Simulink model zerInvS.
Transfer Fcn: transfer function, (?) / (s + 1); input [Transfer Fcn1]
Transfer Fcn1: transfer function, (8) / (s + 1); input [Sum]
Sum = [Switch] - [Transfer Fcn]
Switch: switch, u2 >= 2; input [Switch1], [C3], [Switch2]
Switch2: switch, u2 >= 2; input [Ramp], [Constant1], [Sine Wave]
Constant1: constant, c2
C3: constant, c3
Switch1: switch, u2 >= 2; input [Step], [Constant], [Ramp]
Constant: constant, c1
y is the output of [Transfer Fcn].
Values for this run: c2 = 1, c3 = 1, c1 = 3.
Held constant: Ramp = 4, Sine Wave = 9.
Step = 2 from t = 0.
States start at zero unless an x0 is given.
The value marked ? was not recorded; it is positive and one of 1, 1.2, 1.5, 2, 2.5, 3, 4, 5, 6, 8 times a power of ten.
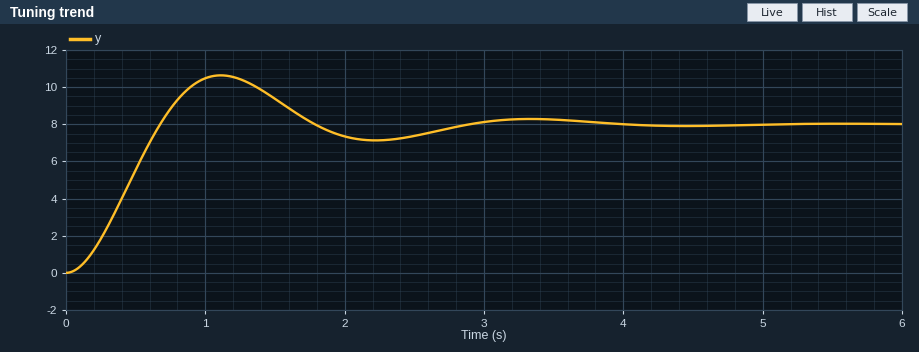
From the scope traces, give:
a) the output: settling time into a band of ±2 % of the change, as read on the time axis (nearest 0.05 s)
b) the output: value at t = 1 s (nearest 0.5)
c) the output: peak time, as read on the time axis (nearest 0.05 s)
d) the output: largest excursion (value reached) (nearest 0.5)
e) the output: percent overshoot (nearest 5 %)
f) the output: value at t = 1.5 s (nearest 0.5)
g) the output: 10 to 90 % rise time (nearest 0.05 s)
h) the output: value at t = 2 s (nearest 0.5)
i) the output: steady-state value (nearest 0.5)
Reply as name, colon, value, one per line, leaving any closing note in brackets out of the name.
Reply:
the output: settling time into a band of ±2 % of the change, as read on the time axis: 3.70 s
the output: value at t = 1 s: 10.5
the output: peak time, as read on the time axis: 1.10 s
the output: largest excursion (value reached): 10.5
the output: percent overshoot: 35 %
the output: value at t = 1.5 s: 9.5
the output: 10 to 90 % rise time: 0.45 s
the output: value at t = 2 s: 7.5
the output: steady-state value: 8.0
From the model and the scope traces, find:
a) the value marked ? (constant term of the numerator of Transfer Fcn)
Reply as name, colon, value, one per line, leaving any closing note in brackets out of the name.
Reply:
the value marked ?: 1
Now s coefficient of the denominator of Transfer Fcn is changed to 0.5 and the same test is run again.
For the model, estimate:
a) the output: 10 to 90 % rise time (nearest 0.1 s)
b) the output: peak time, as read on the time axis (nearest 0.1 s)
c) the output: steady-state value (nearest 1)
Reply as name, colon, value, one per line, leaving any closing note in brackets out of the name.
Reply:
the output: 10 to 90 % rise time: 0.3 s
the output: peak time, as read on the time axis: 0.8 s
the output: steady-state value: 8
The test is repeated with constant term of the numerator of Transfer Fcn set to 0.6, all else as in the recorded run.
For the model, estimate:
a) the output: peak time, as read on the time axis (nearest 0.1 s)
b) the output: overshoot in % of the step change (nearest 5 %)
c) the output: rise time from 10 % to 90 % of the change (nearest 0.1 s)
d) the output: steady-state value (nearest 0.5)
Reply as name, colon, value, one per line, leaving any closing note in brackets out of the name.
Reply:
the output: peak time, as read on the time axis: 1.4 s
the output: overshoot in % of the step change: 25 %
the output: rise time from 10 % to 90 % of the change: 0.6 s
the output: steady-state value: 7.5
